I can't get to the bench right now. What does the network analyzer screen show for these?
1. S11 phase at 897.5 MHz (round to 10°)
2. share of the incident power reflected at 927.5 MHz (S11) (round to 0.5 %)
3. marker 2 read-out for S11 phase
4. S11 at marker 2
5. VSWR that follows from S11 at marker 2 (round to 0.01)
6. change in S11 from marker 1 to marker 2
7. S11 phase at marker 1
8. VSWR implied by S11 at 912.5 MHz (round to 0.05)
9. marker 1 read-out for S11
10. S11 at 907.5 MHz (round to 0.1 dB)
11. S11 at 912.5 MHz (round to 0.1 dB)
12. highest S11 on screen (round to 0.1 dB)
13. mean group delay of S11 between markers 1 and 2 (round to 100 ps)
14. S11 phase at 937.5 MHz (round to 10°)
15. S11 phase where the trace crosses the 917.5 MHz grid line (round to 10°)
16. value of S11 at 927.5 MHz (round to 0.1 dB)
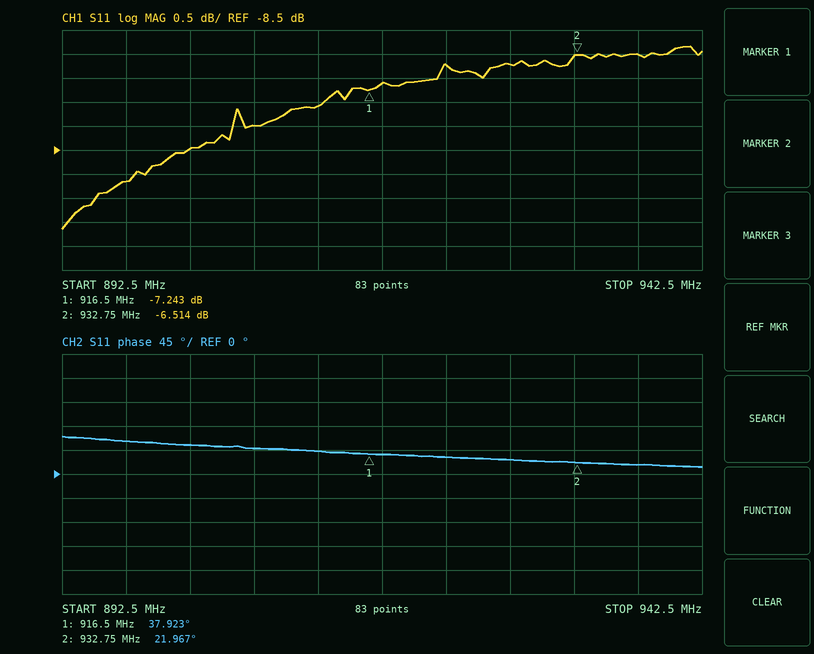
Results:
60°
21.5 %
21.967°
-6.514 dB
2.79
0.729 dB
37.923°
2.45
-7.243 dB
-8.0 dB
-7.6 dB
-6.3 dB
2.7 ns
20°
40°
-6.7 dB
